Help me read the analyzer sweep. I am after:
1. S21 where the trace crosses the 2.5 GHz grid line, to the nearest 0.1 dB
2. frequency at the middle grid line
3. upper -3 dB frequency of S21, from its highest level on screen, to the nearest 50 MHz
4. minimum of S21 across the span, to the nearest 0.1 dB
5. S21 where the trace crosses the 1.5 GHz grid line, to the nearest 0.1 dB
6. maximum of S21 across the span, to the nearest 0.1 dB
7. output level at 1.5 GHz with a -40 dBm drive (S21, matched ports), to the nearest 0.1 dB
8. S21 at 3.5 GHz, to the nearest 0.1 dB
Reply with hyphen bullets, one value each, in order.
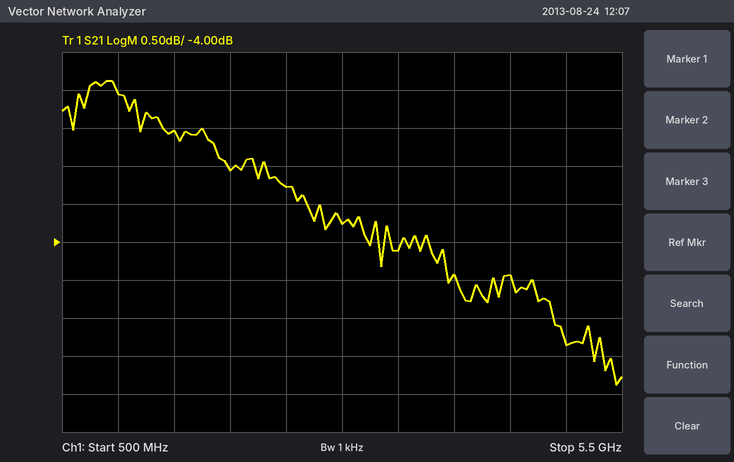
- -3.3 dB
- 3 GHz
- 4.85 GHz
- -5.9 dB
- -2.5 dB
- -1.9 dB
- -42.5 dBm
- -4.1 dB
